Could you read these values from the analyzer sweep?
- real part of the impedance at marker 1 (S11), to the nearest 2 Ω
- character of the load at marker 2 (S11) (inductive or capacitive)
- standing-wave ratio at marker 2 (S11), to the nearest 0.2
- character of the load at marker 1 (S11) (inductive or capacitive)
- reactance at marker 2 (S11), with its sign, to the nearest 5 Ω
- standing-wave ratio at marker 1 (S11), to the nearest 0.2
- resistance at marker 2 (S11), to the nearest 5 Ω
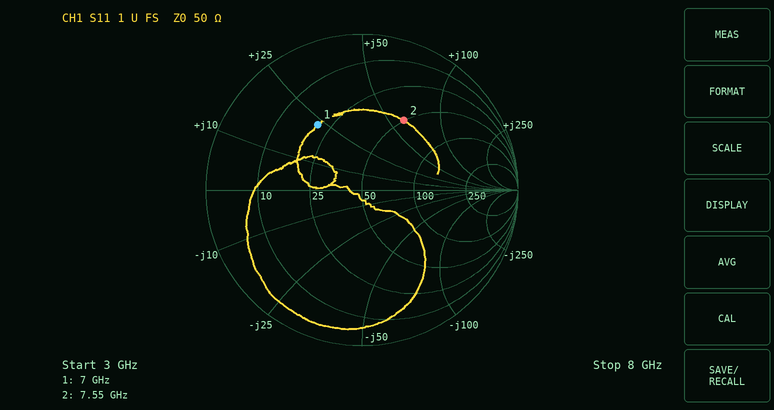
20 Ω
inductive
3.2
inductive
+60 Ω
3.0
50 Ω
